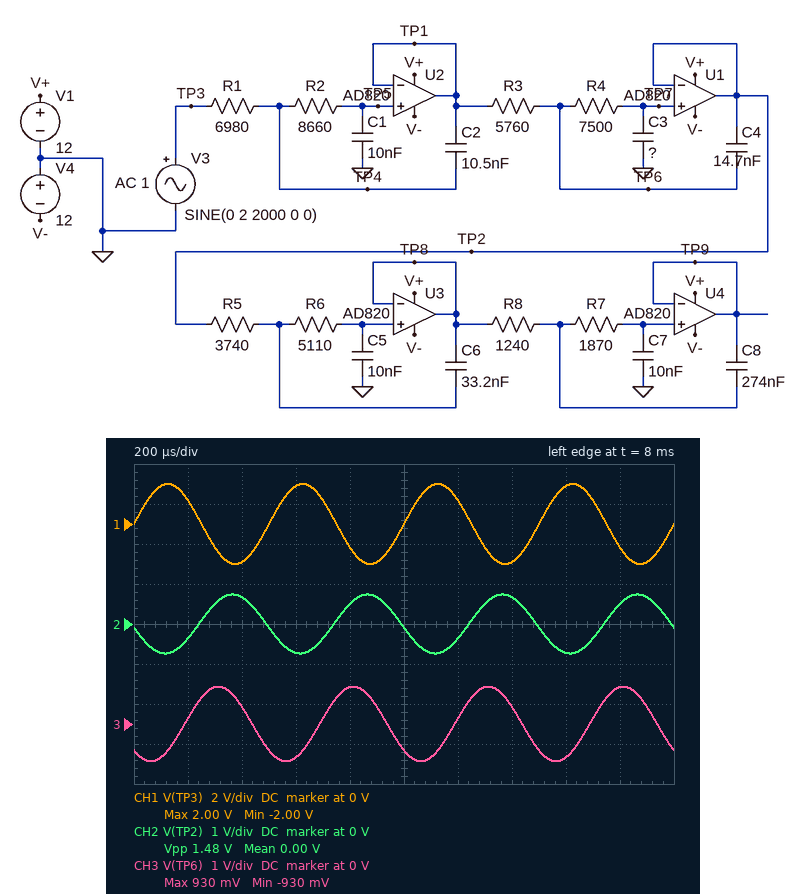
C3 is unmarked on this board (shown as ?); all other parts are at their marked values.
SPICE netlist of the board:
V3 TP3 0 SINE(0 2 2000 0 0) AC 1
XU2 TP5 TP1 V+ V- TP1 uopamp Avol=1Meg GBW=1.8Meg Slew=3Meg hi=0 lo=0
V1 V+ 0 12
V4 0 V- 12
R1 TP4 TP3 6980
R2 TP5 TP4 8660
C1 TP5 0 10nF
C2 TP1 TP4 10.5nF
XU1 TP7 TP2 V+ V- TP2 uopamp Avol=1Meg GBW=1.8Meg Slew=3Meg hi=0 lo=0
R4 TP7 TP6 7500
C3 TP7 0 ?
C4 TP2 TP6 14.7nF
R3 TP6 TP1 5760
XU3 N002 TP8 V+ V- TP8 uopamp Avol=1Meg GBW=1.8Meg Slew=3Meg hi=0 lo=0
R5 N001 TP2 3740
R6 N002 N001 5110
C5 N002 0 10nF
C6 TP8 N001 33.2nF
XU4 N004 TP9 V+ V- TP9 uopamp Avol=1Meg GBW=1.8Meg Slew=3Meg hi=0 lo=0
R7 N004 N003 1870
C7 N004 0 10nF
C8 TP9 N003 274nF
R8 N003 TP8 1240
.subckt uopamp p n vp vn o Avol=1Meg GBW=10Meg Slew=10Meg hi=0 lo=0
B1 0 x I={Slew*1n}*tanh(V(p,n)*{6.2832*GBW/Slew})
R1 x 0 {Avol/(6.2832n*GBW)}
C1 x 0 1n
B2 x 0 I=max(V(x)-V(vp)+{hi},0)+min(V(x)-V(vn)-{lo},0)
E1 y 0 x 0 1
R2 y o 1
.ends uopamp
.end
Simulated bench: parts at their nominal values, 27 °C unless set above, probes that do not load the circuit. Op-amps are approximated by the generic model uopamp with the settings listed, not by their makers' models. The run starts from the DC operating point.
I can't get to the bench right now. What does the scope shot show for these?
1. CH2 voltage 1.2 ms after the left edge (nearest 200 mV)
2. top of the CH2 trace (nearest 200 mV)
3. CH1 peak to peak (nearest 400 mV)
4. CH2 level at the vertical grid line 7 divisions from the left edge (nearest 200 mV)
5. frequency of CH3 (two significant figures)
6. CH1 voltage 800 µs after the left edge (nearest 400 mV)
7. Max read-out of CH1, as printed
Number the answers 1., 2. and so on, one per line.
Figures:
1. -400 mV
2. 800 mV
3. 4.0 V
4. 600 mV
5. 2.0 kHz
6. -1.2 V
7. 2.00 V
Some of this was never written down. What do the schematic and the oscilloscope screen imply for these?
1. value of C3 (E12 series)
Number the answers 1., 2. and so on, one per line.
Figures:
1. 8.2 nF
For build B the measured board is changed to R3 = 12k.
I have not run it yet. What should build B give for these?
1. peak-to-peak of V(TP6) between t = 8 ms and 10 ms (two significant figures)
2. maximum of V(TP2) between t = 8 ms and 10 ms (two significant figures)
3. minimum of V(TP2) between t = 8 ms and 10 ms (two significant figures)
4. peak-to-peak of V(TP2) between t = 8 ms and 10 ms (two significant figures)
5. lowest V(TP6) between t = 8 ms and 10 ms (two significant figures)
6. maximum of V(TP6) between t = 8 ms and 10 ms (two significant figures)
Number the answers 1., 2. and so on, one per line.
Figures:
1. 1.2 V
2. 480 mV
3. -480 mV
4. 950 mV
5. -600 mV
6. 600 mV
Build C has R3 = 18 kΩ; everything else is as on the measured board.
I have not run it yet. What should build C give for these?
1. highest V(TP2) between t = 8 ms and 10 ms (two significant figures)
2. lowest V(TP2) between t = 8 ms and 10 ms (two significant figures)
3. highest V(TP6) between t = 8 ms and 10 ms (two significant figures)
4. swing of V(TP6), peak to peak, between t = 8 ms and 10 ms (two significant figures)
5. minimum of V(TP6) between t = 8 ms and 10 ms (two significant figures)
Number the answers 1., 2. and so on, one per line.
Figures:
1. 330 mV
2. -330 mV
3. 420 mV
4. 840 mV
5. -420 mV
